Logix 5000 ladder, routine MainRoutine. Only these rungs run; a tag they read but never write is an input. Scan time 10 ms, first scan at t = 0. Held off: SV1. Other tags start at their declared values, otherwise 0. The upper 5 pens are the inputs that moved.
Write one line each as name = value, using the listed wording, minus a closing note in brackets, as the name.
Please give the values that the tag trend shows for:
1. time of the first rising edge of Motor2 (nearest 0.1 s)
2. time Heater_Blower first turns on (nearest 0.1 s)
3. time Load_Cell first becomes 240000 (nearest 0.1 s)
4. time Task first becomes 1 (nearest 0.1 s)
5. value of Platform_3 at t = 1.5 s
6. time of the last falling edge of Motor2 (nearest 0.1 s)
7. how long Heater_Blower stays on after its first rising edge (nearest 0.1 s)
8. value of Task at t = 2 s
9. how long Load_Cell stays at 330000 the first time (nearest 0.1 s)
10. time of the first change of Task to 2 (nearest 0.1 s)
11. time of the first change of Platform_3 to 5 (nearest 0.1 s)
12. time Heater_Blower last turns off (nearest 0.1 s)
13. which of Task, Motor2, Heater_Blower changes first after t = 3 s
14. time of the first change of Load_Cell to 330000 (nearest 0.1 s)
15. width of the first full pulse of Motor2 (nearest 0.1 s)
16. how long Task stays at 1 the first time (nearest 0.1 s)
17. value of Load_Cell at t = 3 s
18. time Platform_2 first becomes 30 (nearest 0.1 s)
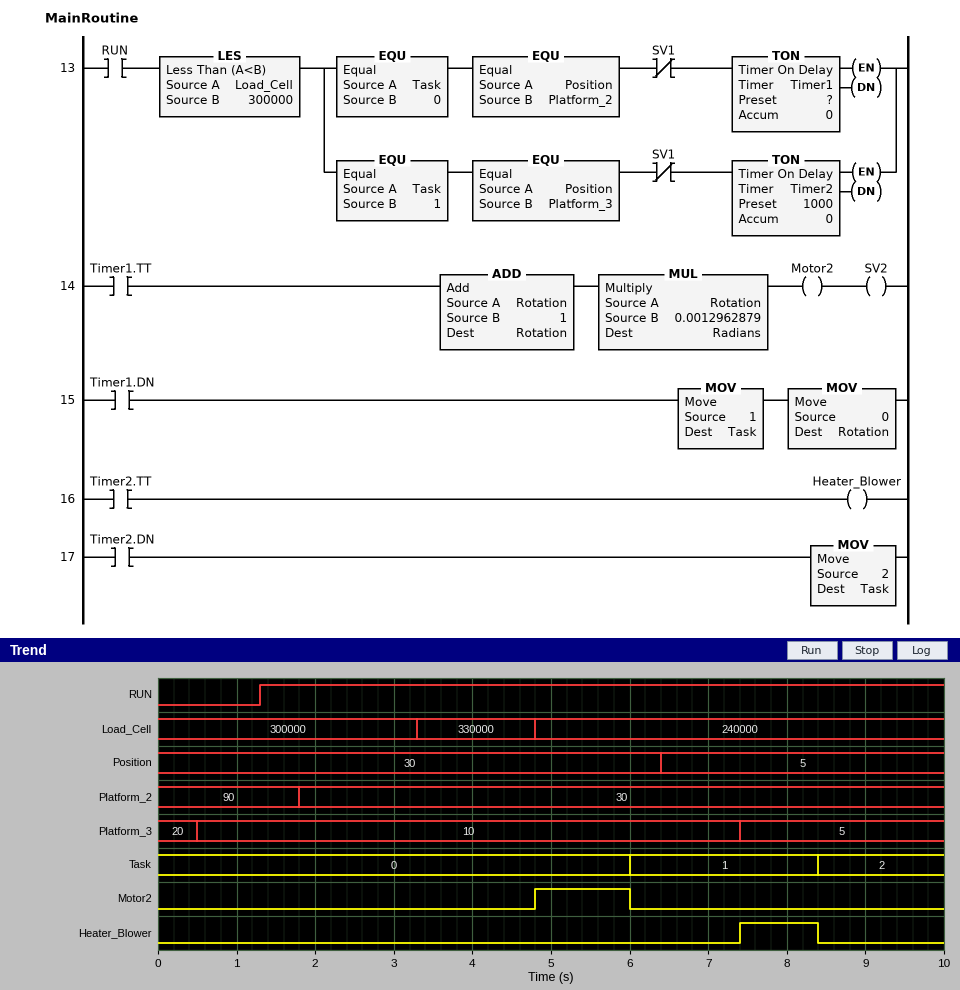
time of the first rising edge of Motor2 = 4.8 s
time Heater_Blower first turns on = 7.4 s
time Load_Cell first becomes 240000 = 4.8 s
time Task first becomes 1 = 6.0 s
value of Platform_3 at t = 1.5 s = 10
time of the last falling edge of Motor2 = 6.0 s
how long Heater_Blower stays on after its first rising edge = 1.0 s
value of Task at t = 2 s = 0
how long Load_Cell stays at 330000 the first time = 1.5 s
time of the first change of Task to 2 = 8.4 s
time of the first change of Platform_3 to 5 = 7.4 s
time Heater_Blower last turns off = 8.4 s
which of Task, Motor2, Heater_Blower changes first after t = 3 s = Motor2
time of the first change of Load_Cell to 330000 = 3.3 s
width of the first full pulse of Motor2 = 1.2 s
how long Task stays at 1 the first time = 2.4 s
value of Load_Cell at t = 3 s = 300000
time Platform_2 first becomes 30 = 1.8 s
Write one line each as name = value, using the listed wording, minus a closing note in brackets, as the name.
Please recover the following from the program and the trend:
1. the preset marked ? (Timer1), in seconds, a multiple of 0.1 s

the preset marked ? (Timer1), in seconds, a multiple of 0.1 s = 1.2 s
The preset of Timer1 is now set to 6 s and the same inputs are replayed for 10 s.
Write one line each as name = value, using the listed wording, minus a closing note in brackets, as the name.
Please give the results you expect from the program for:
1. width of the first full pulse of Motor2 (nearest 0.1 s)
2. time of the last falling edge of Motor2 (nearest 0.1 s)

width of the first full pulse of Motor2 = 1.6 s
time of the last falling edge of Motor2 = 6.4 s
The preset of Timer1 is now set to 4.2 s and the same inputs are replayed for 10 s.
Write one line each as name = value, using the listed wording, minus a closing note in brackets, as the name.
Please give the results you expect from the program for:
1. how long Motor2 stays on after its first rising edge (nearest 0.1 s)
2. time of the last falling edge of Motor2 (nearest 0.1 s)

how long Motor2 stays on after its first rising edge = 1.6 s
time of the last falling edge of Motor2 = 6.4 s
